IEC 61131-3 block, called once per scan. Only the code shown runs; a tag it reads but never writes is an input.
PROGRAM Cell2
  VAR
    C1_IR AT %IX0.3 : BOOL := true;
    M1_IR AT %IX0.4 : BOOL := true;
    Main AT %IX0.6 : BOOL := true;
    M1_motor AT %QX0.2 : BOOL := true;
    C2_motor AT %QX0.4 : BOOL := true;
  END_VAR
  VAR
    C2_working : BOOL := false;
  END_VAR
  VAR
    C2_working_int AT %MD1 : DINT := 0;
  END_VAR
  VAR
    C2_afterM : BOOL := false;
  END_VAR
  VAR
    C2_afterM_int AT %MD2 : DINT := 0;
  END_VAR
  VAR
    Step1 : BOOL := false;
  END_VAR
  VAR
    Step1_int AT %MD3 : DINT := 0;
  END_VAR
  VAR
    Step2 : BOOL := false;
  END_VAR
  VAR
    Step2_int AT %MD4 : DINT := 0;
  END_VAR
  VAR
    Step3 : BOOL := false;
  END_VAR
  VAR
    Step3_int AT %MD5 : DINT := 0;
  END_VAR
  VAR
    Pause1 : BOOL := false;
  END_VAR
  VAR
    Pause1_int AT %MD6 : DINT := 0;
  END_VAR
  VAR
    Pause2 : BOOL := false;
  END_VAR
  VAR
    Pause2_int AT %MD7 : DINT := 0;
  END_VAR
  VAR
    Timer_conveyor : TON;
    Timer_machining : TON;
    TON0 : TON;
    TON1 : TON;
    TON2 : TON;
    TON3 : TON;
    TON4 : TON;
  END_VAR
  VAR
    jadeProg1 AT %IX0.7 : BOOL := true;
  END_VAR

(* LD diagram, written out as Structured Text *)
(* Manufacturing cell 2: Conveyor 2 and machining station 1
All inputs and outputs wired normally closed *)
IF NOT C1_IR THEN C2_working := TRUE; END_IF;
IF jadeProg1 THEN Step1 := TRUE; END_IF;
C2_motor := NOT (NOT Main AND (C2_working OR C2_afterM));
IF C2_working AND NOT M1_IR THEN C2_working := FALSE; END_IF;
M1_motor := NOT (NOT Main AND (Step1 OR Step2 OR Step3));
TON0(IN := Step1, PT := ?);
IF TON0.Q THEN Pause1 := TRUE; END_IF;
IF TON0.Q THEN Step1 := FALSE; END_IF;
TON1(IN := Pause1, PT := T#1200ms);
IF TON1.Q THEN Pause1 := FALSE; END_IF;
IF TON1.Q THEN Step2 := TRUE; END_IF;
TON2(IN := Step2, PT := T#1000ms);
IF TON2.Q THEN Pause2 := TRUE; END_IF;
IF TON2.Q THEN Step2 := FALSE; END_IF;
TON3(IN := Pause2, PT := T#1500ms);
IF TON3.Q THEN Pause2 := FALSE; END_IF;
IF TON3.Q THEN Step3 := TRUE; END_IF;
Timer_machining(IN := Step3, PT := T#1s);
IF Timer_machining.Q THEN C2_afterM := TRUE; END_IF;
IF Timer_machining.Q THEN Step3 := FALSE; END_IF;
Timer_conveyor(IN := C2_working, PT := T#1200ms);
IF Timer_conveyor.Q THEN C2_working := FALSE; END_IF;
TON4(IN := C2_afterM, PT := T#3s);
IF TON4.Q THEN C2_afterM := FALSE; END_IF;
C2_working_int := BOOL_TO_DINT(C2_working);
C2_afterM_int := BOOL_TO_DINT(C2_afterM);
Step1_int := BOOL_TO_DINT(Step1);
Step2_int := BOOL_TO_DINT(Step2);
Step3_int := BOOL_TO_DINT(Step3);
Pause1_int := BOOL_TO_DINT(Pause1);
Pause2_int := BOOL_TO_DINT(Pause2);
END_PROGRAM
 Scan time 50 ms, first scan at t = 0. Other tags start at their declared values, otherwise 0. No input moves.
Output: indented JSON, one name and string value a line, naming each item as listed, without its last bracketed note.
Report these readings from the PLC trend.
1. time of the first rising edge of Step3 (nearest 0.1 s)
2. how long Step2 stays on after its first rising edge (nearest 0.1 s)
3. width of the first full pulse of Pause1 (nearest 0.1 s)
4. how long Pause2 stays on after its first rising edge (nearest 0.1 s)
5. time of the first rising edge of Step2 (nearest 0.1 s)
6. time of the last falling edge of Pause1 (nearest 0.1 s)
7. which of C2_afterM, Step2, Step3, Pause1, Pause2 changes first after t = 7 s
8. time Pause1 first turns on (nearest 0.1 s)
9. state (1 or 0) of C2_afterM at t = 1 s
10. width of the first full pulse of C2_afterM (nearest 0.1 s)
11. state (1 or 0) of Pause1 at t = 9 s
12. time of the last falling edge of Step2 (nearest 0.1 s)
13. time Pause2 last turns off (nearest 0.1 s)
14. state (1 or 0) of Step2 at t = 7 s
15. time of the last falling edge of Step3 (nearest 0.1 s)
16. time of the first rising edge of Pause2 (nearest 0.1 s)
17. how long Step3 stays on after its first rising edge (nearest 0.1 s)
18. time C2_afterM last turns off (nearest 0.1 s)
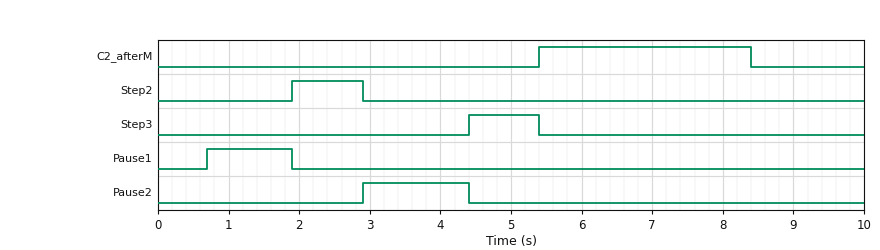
{
  "time of the first rising edge of Step3": "4.4 s",
  "how long Step2 stays on after its first rising edge": "1.0 s",
  "width of the first full pulse of Pause1": "1.2 s",
  "how long Pause2 stays on after its first rising edge": "1.5 s",
  "time of the first rising edge of Step2": "1.9 s",
  "time of the last falling edge of Pause1": "1.9 s",
  "which of C2_afterM, Step2, Step3, Pause1, Pause2 changes first after t = 7 s": "C2_afterM",
  "time Pause1 first turns on": "0.7 s",
  "state (1 or 0) of C2_afterM at t = 1 s": "0",
  "width of the first full pulse of C2_afterM": "3.0 s",
  "state (1 or 0) of Pause1 at t = 9 s": "0",
  "time of the last falling edge of Step2": "2.9 s",
  "time Pause2 last turns off": "4.4 s",
  "state (1 or 0) of Step2 at t = 7 s": "0",
  "time of the last falling edge of Step3": "5.4 s",
  "time of the first rising edge of Pause2": "2.9 s",
  "how long Step3 stays on after its first rising edge": "1.0 s",
  "time C2_afterM last turns off": "8.4 s"
}
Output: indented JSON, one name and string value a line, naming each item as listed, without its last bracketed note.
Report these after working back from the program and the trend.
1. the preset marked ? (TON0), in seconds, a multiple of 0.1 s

{
  "the preset marked ? (TON0), in seconds, a multiple of 0.1 s": "0.7 s"
}
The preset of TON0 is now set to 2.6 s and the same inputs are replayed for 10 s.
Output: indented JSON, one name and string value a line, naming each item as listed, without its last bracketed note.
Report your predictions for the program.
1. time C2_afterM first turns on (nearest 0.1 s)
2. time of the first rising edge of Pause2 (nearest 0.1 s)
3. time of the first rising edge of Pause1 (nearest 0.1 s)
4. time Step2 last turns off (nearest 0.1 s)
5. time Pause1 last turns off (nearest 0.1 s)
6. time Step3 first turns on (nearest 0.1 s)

{
  "time C2_afterM first turns on": "7.3 s",
  "time of the first rising edge of Pause2": "4.8 s",
  "time of the first rising edge of Pause1": "2.6 s",
  "time Step2 last turns off": "4.8 s",
  "time Pause1 last turns off": "3.8 s",
  "time Step3 first turns on": "6.3 s"
}
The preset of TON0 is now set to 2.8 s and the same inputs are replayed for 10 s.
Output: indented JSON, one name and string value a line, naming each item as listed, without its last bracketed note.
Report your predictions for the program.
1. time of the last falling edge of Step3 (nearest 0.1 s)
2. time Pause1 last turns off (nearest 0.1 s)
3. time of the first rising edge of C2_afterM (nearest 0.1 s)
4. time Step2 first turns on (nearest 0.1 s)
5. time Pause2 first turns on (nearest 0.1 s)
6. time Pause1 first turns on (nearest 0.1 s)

{
  "time of the last falling edge of Step3": "7.5 s",
  "time Pause1 last turns off": "4.0 s",
  "time of the first rising edge of C2_afterM": "7.5 s",
  "time Step2 first turns on": "4.0 s",
  "time Pause2 first turns on": "5.0 s",
  "time Pause1 first turns on": "2.8 s"
}
